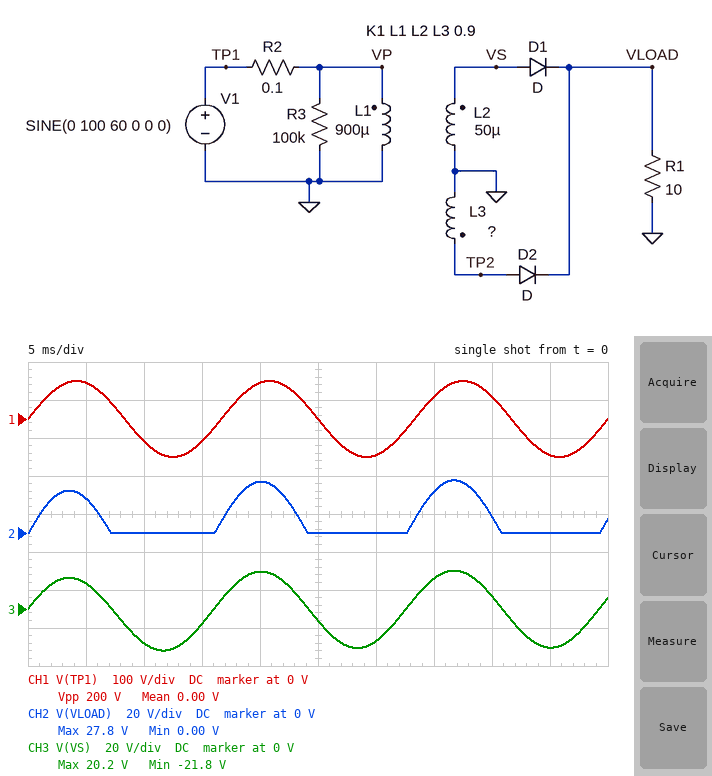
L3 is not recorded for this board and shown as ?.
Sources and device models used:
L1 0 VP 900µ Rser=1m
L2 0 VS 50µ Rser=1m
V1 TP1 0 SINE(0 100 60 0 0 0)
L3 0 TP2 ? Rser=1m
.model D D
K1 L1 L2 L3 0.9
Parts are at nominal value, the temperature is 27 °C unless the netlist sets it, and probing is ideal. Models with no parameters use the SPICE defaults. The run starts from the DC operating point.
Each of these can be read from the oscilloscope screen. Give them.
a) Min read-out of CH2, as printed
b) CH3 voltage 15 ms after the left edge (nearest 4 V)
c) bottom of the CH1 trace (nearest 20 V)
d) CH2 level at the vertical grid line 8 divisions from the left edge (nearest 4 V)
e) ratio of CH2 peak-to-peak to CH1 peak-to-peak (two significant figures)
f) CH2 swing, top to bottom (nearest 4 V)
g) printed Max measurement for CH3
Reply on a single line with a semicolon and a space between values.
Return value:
0.00 V; -8 V; -100 V; 8 V; 0.14; 28 V; 20.2 V
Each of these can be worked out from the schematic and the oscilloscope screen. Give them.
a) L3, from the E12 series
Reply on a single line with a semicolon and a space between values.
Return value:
100 µH
